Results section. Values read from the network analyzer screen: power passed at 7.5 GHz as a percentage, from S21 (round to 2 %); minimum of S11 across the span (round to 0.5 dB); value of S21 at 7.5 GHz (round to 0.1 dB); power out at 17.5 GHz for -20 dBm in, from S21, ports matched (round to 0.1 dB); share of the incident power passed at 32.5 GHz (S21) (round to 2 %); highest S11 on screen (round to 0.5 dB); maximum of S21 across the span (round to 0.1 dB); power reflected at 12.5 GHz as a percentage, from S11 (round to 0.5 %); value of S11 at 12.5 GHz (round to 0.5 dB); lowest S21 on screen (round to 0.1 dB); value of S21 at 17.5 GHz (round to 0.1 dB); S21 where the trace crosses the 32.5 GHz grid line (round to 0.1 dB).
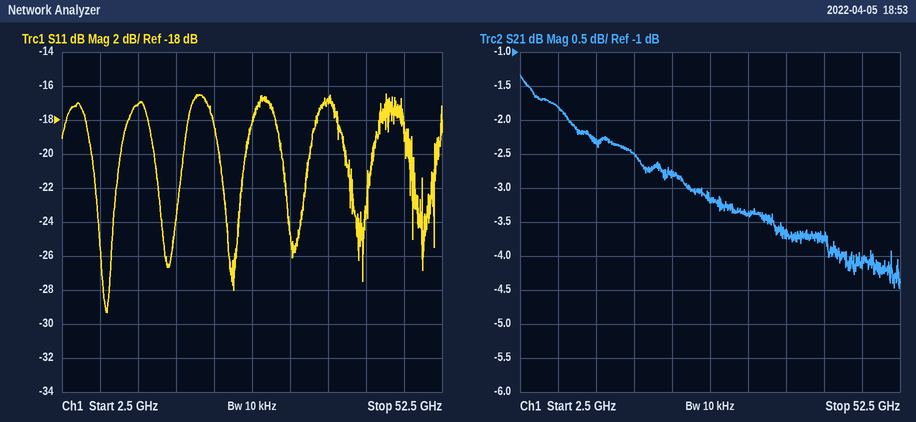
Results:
66 %
-29.5 dB
-1.8 dB
-22.5 dBm
46 %
-16.5 dB
-1.3 dB
2.0 %
-17.0 dB
-4.5 dB
-2.5 dB
-3.4 dB
